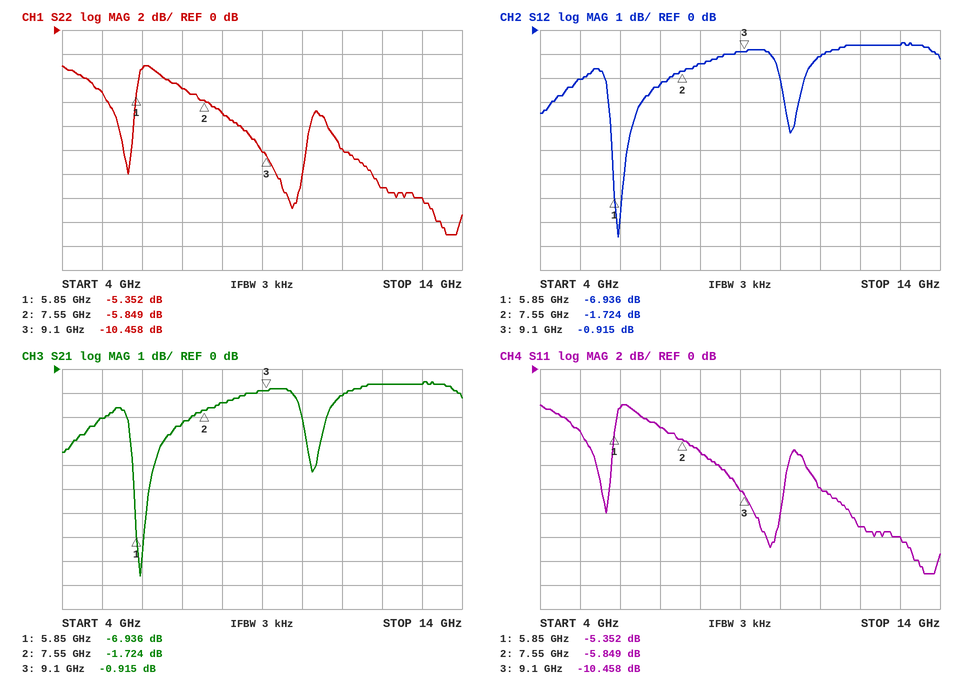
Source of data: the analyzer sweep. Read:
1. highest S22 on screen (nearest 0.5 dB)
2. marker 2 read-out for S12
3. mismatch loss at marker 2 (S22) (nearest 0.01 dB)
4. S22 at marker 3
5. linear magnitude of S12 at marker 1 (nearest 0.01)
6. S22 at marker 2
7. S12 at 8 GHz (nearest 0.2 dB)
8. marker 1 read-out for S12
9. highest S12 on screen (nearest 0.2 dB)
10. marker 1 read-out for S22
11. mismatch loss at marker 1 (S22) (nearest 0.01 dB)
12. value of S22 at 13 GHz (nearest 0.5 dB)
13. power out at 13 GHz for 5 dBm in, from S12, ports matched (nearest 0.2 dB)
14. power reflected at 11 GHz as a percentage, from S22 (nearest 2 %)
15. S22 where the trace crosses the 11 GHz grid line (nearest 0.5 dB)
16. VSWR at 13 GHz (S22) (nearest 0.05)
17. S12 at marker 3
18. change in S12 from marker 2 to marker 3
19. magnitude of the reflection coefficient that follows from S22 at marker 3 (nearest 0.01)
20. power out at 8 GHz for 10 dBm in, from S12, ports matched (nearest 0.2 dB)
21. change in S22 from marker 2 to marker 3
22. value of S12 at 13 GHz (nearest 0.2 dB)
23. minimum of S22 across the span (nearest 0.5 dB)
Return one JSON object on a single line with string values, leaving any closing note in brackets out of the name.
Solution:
{"highest S22 on screen": "-3.0 dB", "marker 2 read-out for S12": "-1.724 dB", "mismatch loss at marker 2 (S22)": "1.31 dB", "S22 at marker 3": "-10.458 dB", "linear magnitude of S12 at marker 1": "0.45", "S22 at marker 2": "-5.849 dB", "S12 at 8 GHz": "-1.4 dB", "marker 1 read-out for S12": "-6.936 dB", "highest S12 on screen": "-0.6 dB", "marker 1 read-out for S22": "-5.352 dB", "mismatch loss at marker 1 (S22)": "1.50 dB", "value of S22 at 13 GHz": "-14.0 dB", "power out at 13 GHz for 5 dBm in, from S12, ports matched": "4.4 dBm", "power reflected at 11 GHz as a percentage, from S22": "10 %", "S22 where the trace crosses the 11 GHz grid line": "-10.0 dB", "VSWR at 13 GHz (S22)": "1.50", "S12 at marker 3": "-0.915 dB", "change in S12 from marker 2 to marker 3": "0.809 dB", "magnitude of the reflection coefficient that follows from S22 at marker 3": "0.30", "power out at 8 GHz for 10 dBm in, from S12, ports matched": "8.6 dBm", "change in S22 from marker 2 to marker 3": "-4.609 dB", "value of S12 at 13 GHz": "-0.6 dB", "minimum of S22 across the span": "-17.0 dB"}
